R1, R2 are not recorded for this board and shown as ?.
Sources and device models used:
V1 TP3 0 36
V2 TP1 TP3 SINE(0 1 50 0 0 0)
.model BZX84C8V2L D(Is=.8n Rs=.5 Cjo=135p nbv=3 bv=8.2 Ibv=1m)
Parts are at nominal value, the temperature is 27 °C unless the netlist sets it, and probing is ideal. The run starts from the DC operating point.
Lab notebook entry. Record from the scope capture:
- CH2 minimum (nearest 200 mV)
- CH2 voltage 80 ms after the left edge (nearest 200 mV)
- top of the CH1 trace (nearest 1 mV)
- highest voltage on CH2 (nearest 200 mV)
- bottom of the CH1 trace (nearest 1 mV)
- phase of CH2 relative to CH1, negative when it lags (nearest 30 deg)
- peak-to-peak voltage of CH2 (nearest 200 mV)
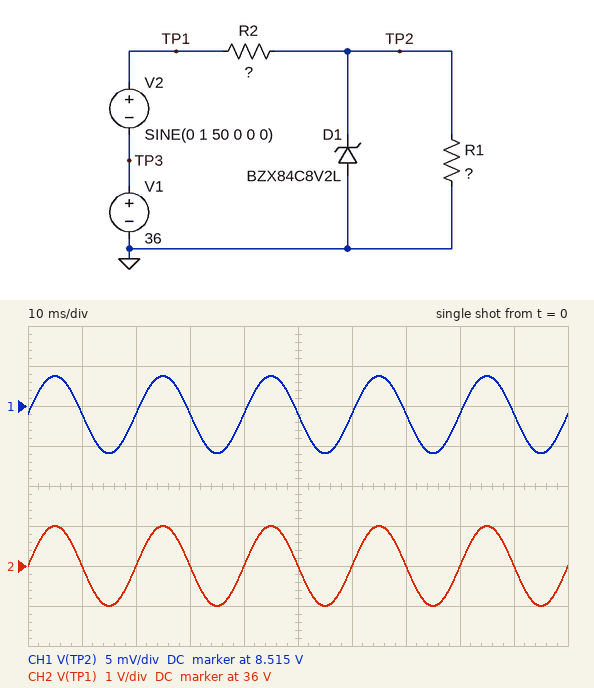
35.0 V
36.0 V
8.519 V
37.0 V
8.509 V
0 deg
2.0 V
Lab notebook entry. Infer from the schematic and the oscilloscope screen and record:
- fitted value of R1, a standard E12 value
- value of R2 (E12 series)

560 Ω
470 Ω
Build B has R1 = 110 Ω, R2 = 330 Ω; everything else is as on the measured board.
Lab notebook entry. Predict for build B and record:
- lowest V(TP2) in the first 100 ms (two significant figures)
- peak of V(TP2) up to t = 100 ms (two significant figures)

8.3 V
8.4 V
